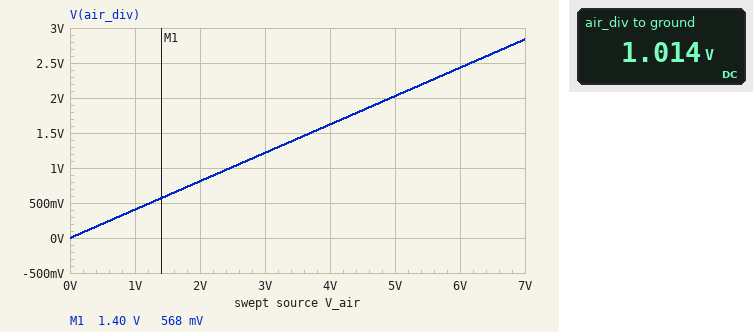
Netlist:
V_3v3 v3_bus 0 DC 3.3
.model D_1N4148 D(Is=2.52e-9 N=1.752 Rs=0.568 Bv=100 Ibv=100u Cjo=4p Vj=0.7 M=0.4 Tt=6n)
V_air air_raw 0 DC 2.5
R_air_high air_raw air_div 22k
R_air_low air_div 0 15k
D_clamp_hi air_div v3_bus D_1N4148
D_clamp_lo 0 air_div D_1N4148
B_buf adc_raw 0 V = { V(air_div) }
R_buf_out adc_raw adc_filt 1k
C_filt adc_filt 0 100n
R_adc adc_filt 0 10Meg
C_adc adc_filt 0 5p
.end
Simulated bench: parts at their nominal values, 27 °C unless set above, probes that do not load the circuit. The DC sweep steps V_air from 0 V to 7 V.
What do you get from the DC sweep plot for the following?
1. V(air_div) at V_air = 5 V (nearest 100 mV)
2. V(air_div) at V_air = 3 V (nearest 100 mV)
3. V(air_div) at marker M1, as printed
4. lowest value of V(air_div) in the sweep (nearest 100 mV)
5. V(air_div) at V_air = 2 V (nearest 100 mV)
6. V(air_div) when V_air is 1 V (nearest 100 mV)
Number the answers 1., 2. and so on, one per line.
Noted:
1. 2.0 V
2. 1.2 V
3. 568 mV
4. 0 V
5. 800 mV
6. 400 mV
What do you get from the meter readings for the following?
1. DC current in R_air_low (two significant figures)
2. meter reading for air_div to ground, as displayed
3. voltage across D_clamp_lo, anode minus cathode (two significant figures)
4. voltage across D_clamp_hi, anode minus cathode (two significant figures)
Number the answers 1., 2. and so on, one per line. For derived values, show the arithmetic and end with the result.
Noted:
1. (1.014 V) / 15 kΩ = 68 µA
2. 1.014 V
3. 0 V - 1.014 V = -1.0 V
4. 1.014 V - 3.3 V = -2.3 V
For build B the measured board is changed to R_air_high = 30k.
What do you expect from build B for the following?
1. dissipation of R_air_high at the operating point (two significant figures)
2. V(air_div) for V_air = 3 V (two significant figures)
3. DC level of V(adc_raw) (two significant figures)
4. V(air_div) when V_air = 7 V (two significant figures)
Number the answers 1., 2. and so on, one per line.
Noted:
1. 93 µW
2. 1.0 V
3. 830 mV
4. 2.3 V
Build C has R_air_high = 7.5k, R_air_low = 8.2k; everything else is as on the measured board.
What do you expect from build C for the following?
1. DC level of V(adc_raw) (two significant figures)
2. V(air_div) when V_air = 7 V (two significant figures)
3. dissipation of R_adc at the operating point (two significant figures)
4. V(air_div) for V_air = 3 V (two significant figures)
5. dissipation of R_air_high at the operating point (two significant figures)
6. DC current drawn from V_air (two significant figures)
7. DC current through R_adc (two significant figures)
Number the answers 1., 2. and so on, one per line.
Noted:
1. 1.3 V
2. 3.6 V
3. 170 nW
4. 1.6 V
5. 190 µW
6. 160 µA
7. 130 nA
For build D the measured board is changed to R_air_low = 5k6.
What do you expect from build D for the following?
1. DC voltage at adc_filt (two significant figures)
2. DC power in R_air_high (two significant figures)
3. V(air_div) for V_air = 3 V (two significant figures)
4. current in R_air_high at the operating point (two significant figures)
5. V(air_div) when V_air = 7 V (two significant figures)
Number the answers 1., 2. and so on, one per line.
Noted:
1. 510 mV
2. 180 µW
3. 610 mV
4. 91 µA
5. 1.4 V
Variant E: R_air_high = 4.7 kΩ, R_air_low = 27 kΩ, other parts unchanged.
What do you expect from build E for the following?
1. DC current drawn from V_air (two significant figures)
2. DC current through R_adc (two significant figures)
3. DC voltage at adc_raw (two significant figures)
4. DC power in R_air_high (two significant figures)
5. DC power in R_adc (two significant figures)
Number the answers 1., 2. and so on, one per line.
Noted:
1. 79 µA
2. 210 nA
3. 2.1 V
4. 29 µW
5. 450 nW
